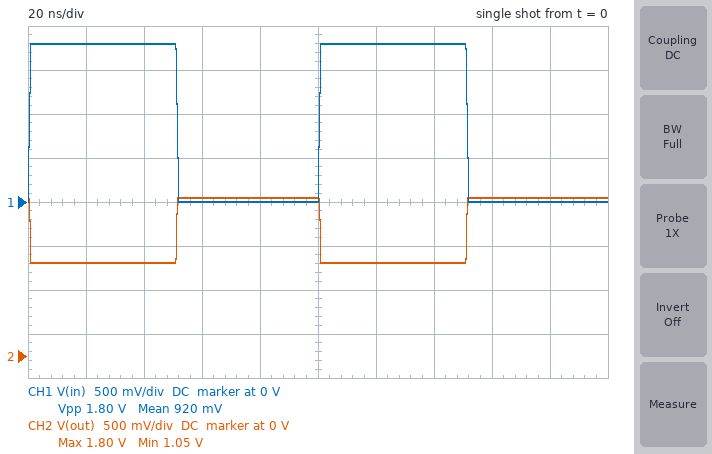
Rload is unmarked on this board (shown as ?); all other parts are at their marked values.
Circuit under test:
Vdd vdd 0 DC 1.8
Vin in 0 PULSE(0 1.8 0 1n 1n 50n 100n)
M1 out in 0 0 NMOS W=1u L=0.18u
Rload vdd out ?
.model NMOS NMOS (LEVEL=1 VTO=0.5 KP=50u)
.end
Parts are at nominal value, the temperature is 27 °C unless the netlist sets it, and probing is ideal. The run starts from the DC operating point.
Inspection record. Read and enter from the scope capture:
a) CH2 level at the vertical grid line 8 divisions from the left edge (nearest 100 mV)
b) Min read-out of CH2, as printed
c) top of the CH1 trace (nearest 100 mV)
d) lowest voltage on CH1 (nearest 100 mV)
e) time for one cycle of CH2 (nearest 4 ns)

1.8 V
1.05 V
1.8 V
0 V
100 ns
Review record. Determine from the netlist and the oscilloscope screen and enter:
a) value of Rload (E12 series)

3.3 kΩ
